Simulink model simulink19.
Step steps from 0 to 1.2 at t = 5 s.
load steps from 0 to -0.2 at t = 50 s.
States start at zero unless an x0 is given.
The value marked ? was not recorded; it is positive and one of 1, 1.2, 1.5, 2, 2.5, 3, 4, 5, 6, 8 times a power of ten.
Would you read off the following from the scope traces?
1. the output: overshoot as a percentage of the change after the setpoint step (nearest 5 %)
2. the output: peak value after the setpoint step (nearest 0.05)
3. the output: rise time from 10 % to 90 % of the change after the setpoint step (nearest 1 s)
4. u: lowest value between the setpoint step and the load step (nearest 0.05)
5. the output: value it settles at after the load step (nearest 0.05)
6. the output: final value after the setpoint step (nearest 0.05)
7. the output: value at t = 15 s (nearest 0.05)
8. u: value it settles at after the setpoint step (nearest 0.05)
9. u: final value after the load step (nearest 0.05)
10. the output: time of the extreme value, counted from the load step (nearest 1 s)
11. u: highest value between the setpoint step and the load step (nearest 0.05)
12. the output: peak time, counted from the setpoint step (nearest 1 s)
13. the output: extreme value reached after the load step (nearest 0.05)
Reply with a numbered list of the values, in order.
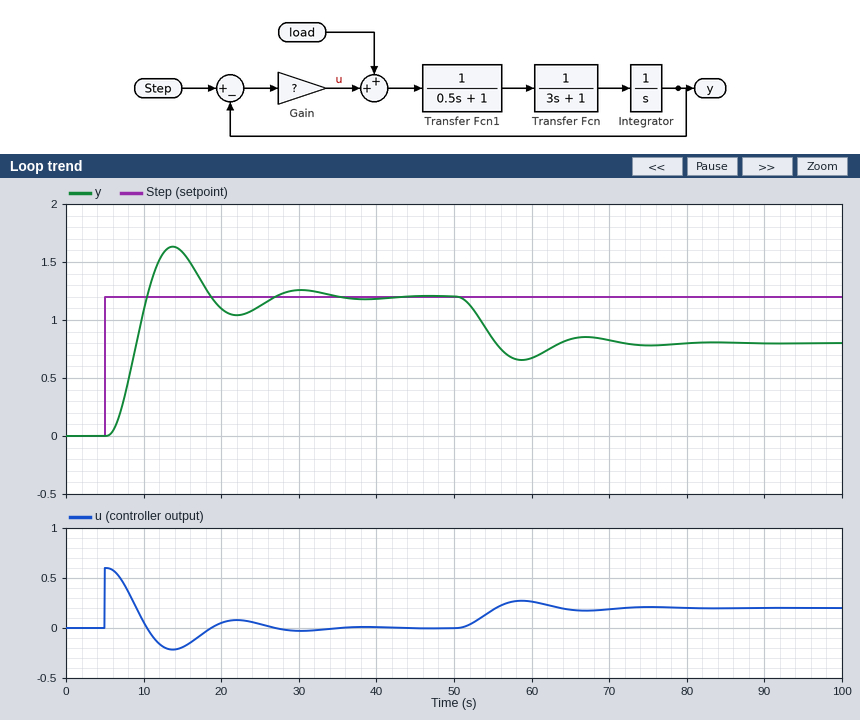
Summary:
1. 35 %
2. 1.65
3. 3 s
4. -0.20
5. 0.80
6. 1.20
7. 1.60
8. 0.00
9. 0.20
10. 9 s
11. 0.60
12. 9 s
13. 0.65
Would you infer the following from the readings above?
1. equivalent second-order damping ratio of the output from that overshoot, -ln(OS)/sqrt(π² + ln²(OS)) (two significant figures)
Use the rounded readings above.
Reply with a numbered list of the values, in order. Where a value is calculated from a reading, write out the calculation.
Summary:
1. ln(0.35) = -1.050; 1.050 / sqrt(9.870 + 1.102) = 0.32
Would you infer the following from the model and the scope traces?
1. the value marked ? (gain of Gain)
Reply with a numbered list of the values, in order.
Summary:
1. 0.5
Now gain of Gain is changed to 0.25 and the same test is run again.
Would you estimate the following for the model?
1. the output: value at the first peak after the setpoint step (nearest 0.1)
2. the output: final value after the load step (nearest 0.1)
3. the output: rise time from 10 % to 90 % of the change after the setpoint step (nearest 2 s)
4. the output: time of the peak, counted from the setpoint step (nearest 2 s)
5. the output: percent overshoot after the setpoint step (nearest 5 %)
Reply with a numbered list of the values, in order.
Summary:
1. 1.4
2. 0.4
3. 6 s
4. 14 s
5. 15 %
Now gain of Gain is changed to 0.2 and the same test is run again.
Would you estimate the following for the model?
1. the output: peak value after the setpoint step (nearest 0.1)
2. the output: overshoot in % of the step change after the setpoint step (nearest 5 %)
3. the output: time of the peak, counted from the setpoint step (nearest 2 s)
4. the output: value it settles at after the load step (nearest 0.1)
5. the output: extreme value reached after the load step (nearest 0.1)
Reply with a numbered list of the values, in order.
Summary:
1. 1.3
2. 10 %
3. 16 s
4. 0.2
5. 0.1
